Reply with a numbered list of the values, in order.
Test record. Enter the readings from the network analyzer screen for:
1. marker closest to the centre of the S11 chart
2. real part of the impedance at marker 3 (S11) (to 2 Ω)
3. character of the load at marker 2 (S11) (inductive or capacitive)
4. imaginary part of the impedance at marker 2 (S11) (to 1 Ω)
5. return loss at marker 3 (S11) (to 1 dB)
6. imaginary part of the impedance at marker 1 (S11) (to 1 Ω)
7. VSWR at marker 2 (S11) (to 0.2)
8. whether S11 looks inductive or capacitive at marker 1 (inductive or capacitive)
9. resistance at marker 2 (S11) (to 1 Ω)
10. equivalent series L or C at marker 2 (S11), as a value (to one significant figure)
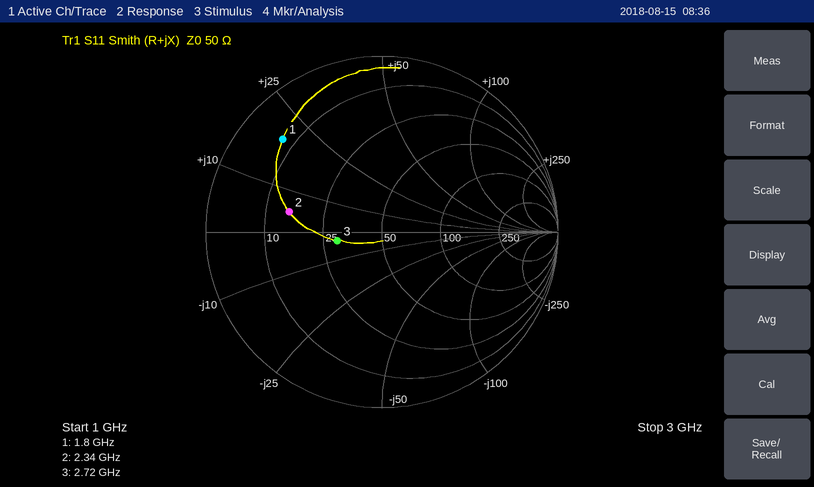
1. marker 3
2. 30 Ω
3. inductive
4. +5 Ω
5. 12 dB
6. +19 Ω
7. 3.4
8. inductive
9. 15 Ω
10. 300 pH
